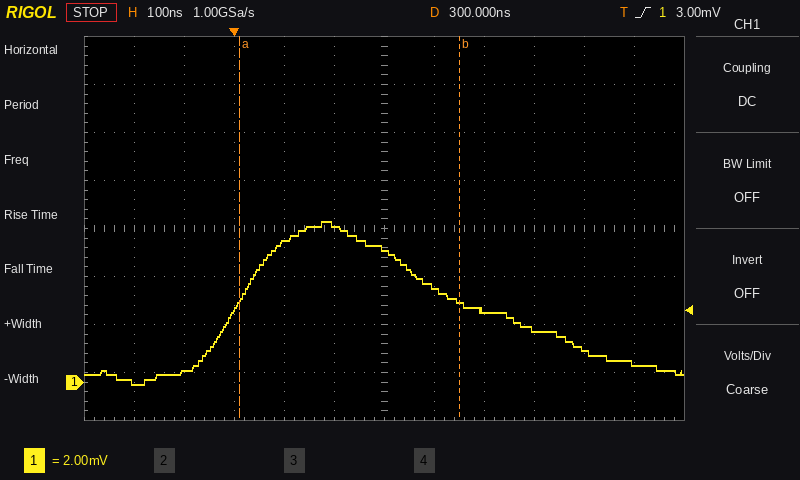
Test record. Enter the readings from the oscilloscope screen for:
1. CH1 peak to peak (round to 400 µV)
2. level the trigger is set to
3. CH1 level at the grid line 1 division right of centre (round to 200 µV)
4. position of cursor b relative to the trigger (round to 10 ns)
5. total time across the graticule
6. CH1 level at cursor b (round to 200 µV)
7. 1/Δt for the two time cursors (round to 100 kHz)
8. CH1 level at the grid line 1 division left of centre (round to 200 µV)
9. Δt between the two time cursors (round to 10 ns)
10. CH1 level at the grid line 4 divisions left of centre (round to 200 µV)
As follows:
6.8 mV
3.00 mV
4.0 mV
+450 ns
1.2 µs
3.4 mV
2.3 MHz
6.6 mV
440 ns
400 µV
